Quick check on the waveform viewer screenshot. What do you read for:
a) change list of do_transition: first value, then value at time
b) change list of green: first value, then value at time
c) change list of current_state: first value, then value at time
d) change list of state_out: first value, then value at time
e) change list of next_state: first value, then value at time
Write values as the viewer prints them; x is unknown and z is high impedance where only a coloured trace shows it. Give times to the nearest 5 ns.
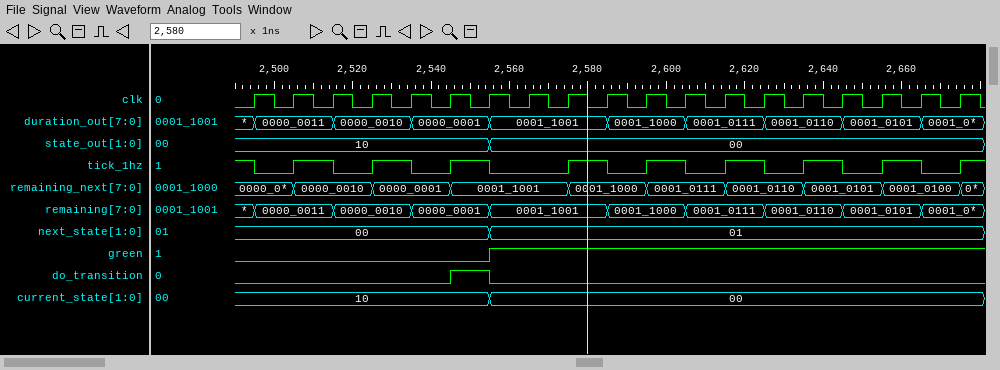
0, 1 at 2545 ns, 0 at 2555 ns
0, 1 at 2555 ns
10, 00 at 2555 ns
10, 00 at 2555 ns
00, 01 at 2555 ns
